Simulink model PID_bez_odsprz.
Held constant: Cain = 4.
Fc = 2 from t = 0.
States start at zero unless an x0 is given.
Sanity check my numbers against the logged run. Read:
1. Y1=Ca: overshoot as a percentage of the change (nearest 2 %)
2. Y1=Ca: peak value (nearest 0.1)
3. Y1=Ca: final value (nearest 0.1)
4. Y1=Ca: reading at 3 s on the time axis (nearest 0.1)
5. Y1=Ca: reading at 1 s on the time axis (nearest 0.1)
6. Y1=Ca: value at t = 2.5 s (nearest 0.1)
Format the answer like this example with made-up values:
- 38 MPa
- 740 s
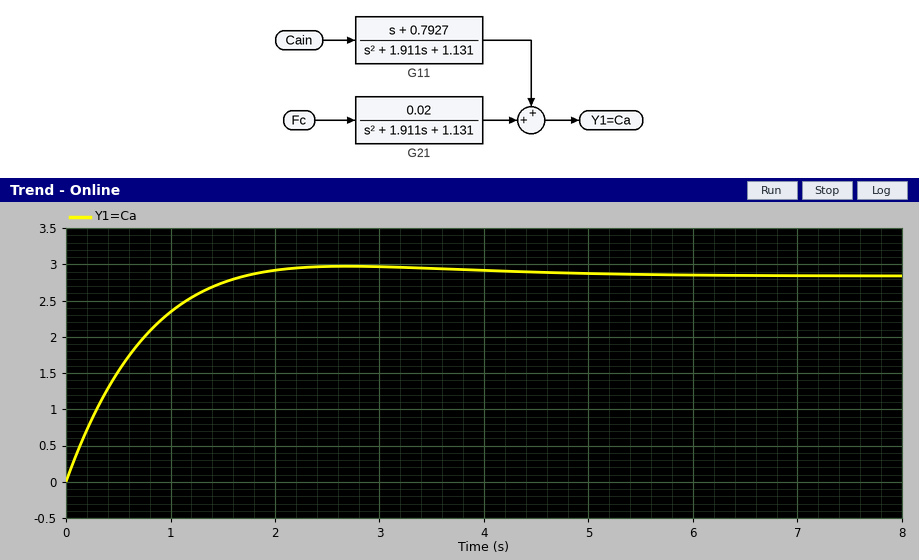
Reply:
- 4 %
- 3.0
- 2.8
- 3.0
- 2.3
- 3.0
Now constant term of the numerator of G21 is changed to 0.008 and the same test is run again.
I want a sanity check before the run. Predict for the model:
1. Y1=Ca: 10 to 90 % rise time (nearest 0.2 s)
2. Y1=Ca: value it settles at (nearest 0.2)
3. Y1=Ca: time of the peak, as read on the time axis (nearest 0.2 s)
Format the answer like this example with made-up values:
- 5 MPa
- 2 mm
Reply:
- 1.2 s
- 2.8
- 2.6 s
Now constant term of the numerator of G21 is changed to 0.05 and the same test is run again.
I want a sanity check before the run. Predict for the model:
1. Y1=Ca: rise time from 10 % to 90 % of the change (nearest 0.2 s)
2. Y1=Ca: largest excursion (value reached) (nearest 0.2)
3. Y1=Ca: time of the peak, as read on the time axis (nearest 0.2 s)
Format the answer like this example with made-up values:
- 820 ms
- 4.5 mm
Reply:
- 1.2 s
- 3.0
- 2.8 s
